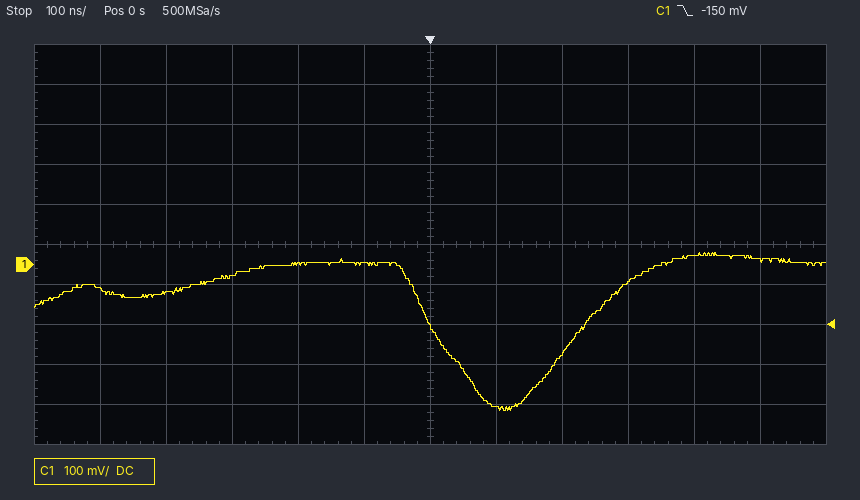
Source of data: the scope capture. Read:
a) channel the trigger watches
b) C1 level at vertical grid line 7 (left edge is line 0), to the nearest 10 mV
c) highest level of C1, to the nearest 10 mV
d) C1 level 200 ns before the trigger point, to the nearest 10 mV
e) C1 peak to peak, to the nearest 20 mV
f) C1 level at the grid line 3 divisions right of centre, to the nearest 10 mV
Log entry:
C1
-360 mV
30 mV
0 mV
400 mV
-40 mV
